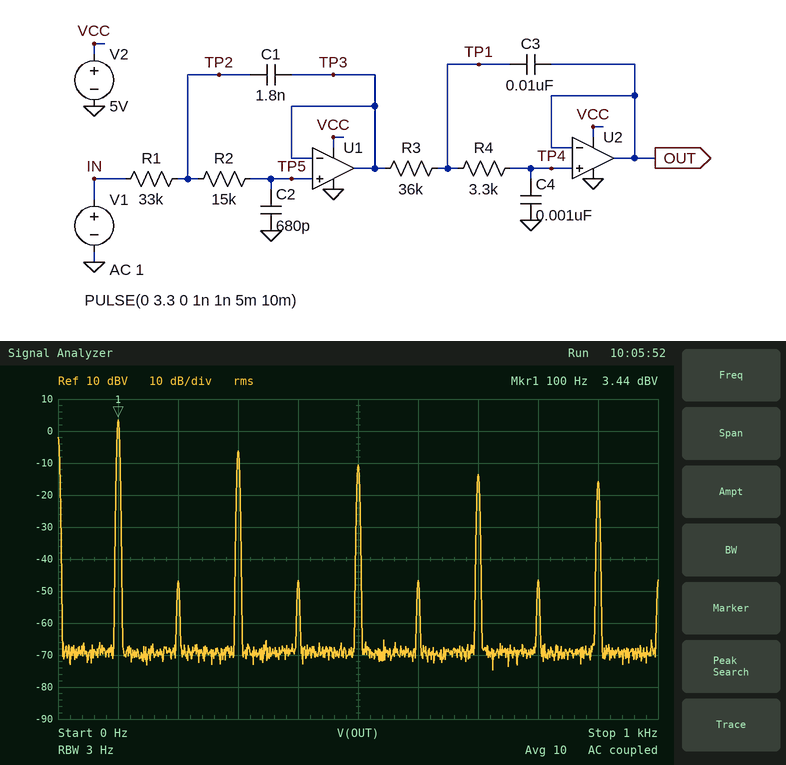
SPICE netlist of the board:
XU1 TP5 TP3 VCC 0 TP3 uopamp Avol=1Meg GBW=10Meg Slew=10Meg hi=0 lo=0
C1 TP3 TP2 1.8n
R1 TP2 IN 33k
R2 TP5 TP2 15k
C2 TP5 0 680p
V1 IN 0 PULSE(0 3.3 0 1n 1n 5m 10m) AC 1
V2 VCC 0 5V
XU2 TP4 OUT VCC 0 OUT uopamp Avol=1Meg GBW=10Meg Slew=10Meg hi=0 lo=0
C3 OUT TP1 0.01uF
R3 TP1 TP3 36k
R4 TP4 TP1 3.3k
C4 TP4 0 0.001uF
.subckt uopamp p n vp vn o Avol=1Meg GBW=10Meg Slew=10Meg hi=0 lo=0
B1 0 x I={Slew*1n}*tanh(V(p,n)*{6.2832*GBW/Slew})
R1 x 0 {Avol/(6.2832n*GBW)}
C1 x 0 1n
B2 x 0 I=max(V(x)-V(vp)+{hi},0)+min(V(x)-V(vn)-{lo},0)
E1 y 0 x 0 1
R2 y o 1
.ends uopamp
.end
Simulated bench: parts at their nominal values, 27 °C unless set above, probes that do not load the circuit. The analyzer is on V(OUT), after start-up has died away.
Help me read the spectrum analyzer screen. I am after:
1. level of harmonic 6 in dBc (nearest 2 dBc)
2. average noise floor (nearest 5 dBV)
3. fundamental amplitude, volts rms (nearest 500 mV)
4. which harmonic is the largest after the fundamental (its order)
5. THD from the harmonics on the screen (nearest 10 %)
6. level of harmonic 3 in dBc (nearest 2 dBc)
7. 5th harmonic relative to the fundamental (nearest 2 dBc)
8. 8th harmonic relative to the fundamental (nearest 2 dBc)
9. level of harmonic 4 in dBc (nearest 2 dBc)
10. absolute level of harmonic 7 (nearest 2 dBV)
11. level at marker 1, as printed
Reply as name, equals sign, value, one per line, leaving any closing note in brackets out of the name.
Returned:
level of harmonic 6 in dBc = -50 dBc
average noise floor = -70 dBV
fundamental amplitude, volts rms = 1.5 V
which harmonic is the largest after the fundamental = 3
THD from the harmonics on the screen = 40 %
level of harmonic 3 in dBc = -10 dBc
5th harmonic relative to the fundamental = -14 dBc
8th harmonic relative to the fundamental = -50 dBc
level of harmonic 4 in dBc = -50 dBc
absolute level of harmonic 7 = -14 dBV
level at marker 1, as printed = 3.44 dBV
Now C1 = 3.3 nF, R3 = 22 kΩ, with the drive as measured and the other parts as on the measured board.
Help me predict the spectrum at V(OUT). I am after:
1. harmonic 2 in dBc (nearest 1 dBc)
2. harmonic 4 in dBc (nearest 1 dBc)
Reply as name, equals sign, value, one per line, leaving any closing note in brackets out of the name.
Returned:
harmonic 2 in dBc = -45 dBc
harmonic 4 in dBc = -45 dBc
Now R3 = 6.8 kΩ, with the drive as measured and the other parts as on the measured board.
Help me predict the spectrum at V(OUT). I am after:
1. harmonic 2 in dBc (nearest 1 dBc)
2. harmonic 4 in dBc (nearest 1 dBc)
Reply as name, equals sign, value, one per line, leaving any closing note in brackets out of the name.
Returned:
harmonic 2 in dBc = -54 dBc
harmonic 4 in dBc = -54 dBc
